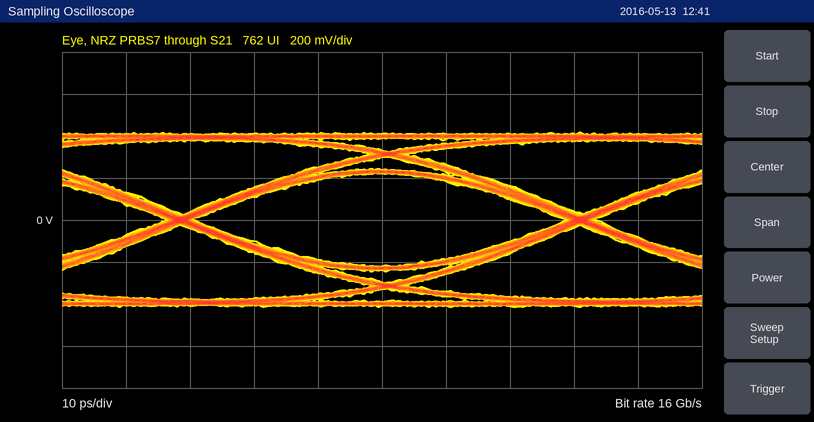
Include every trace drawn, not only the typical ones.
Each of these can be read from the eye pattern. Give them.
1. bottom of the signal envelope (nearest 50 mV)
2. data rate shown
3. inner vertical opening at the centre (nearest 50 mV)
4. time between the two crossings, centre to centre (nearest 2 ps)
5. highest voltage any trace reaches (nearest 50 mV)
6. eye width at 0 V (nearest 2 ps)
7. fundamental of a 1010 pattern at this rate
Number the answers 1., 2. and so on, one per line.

1. -400 mV
2. 16 Gb/s
3. 450 mV
4. 62 ps
5. 400 mV
6. 58 ps
7. 8 GHz
